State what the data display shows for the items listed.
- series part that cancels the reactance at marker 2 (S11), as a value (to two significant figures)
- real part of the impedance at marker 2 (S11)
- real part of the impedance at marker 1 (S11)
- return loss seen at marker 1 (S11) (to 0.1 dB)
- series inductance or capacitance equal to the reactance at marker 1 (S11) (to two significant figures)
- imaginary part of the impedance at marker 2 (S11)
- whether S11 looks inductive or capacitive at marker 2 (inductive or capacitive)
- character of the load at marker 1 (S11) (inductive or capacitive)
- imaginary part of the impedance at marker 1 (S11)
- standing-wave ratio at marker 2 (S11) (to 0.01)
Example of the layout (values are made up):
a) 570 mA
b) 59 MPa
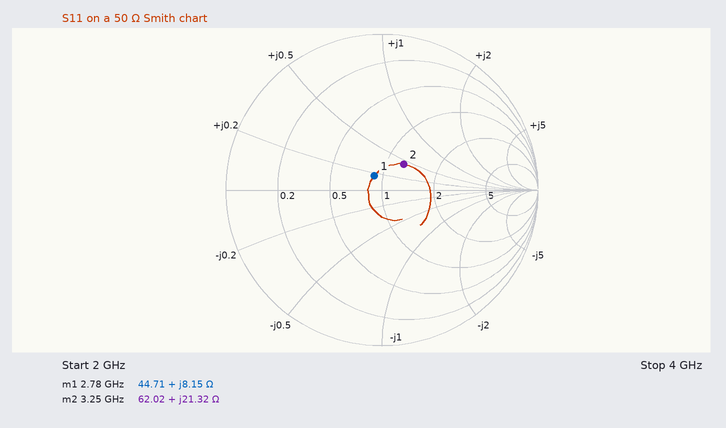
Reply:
a) 2.3 pF
b) 62.02 Ω
c) 44.71 Ω
d) 19.8 dB
e) 470 pH
f) +21.32 Ω
g) inductive
h) inductive
i) +8.15 Ω
j) 1.55
